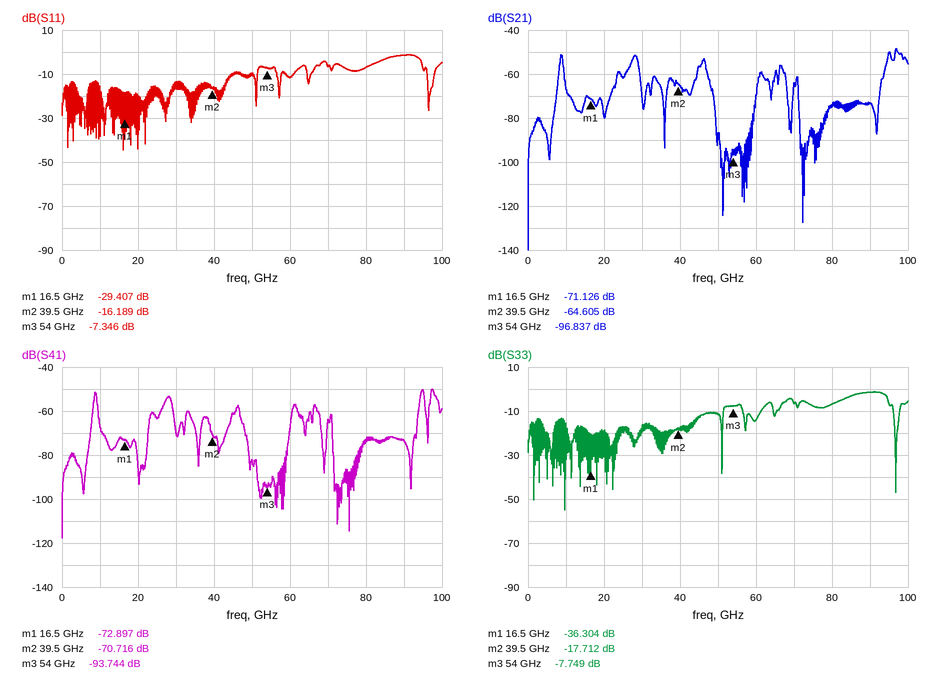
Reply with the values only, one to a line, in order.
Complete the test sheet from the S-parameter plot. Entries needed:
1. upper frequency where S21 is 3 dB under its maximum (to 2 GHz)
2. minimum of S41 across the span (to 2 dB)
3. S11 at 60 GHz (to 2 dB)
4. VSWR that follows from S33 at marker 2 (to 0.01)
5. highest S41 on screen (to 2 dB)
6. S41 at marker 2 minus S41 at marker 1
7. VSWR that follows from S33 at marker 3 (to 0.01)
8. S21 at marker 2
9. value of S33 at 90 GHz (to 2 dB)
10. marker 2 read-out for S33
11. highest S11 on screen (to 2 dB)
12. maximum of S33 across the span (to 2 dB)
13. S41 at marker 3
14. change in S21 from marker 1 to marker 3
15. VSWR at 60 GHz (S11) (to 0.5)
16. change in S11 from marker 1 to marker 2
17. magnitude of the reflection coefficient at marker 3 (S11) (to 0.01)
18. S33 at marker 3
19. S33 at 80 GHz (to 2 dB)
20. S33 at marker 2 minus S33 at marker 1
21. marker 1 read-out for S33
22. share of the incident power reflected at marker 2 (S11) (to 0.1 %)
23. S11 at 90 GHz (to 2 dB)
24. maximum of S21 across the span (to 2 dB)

98 GHz
-118 dB
-12 dB
1.30
-50 dB
2.181 dB
2.39
-64.605 dB
-2 dB
-17.712 dB
-2 dB
-2 dB
-93.744 dB
-25.711 dB
1.5
13.218 dB
0.43
-7.749 dB
-6 dB
18.592 dB
-36.304 dB
2.4 %
-2 dB
-48 dB
